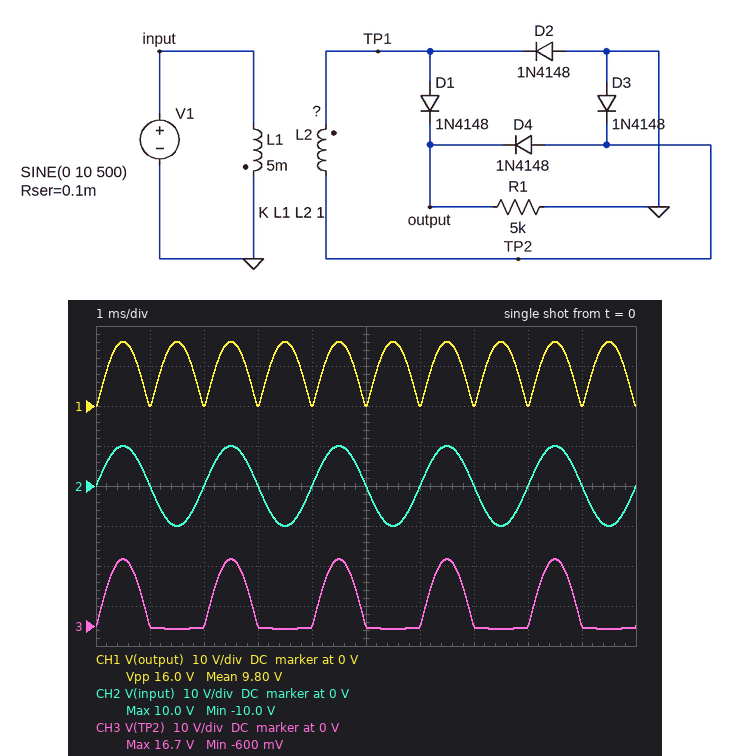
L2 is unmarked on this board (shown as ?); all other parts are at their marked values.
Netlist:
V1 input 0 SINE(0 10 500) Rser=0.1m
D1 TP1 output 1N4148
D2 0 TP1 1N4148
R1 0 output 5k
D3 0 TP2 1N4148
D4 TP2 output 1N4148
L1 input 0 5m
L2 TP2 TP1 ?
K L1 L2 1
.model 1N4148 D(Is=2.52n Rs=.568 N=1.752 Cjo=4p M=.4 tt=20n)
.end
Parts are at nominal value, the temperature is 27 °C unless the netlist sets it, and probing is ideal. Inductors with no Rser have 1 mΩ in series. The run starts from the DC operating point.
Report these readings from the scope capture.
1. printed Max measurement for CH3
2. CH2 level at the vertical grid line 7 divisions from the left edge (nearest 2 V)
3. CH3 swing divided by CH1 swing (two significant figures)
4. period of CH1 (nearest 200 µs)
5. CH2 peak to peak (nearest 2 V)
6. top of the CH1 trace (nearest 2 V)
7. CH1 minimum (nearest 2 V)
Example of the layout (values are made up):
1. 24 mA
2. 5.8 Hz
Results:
1. 16.7 V
2. 0 V
3. 1.1
4. 1.0 ms
5. 20 V
6. 16 V
7. 0 V
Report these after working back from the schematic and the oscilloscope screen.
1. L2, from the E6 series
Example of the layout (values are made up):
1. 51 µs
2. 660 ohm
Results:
1. 15 mH
